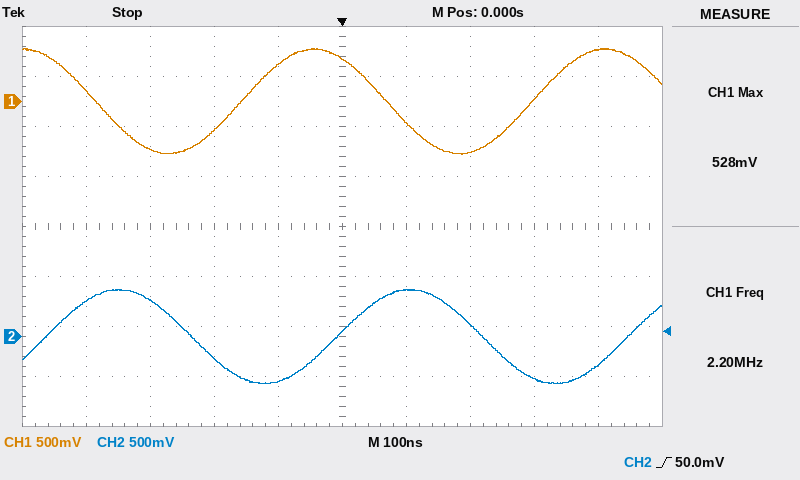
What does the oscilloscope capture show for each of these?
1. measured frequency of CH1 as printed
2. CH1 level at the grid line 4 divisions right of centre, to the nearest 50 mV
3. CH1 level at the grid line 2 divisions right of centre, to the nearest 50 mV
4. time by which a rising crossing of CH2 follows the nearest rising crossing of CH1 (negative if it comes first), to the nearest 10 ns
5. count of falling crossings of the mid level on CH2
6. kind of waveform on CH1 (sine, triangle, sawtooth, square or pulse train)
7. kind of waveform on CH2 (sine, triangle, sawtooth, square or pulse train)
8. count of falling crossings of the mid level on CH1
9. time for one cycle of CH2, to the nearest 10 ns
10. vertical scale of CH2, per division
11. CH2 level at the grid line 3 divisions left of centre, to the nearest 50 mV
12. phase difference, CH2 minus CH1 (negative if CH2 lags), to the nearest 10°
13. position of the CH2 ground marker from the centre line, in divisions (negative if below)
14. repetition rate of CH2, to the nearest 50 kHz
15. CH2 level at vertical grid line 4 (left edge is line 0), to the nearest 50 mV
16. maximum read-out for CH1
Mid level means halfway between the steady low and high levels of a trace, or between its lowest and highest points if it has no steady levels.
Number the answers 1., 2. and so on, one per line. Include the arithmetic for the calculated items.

1. 2.20 MHz
2. 500 mV
3. -500 mV
4. +150 ns
5. 2
6. sine
7. sine
8. 2
9. 450 ns
10. 500 mV
11. 350 mV
12. −360° × (+150 ns) / 450 ns ≈ -120°
13. -2.2 div
14. 1 / 450 ns ≈ 2.22 MHz, so 2.20 MHz to the nearest 50 kHz
15. -450 mV
16. 528 mV
